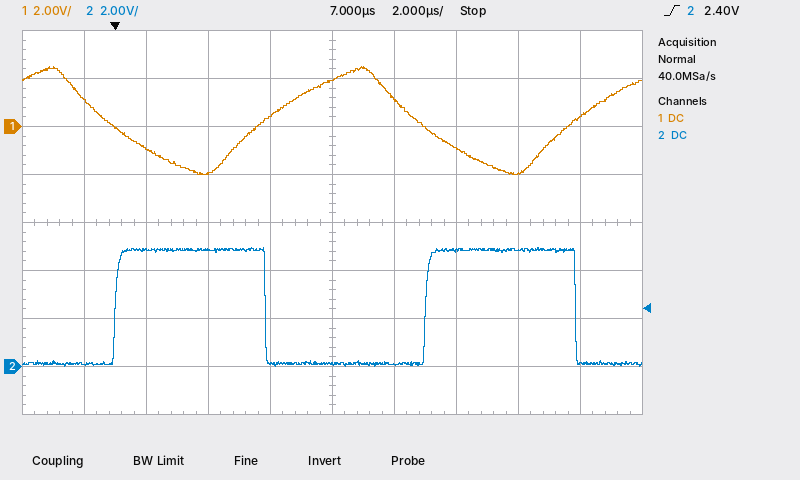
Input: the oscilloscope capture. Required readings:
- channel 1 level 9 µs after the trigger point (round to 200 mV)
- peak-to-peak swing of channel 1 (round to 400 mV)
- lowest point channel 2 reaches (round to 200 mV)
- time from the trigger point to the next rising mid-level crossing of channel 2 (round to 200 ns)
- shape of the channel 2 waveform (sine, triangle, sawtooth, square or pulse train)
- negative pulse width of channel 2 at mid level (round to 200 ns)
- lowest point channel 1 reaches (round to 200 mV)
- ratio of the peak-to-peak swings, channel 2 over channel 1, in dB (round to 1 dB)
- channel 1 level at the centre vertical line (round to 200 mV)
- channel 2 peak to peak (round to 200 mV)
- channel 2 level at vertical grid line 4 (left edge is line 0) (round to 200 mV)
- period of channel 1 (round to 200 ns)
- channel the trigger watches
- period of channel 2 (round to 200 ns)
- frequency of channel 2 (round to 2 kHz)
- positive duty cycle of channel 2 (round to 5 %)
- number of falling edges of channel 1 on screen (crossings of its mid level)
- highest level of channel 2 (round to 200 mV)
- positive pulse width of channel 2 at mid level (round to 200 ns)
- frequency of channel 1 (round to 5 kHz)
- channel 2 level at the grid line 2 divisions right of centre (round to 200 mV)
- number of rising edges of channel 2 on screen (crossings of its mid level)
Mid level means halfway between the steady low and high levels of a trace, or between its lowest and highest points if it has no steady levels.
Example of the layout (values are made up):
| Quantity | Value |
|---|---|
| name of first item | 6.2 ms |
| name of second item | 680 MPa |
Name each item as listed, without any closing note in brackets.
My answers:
| Quantity | Value |
|---|---|
| channel 1 level 9 µs after the trigger point | 1.2 V |
| peak-to-peak swing of channel 1 | 4.4 V |
| lowest point channel 2 reaches | 0.0 V |
| time from the trigger point to the next rising mid-level crossing of channel 2 | 10.0 µs |
| shape of the channel 2 waveform | square |
| negative pulse width of channel 2 at mid level | 5.2 µs |
| lowest point channel 1 reaches | -2.0 V |
| ratio of the peak-to-peak swings, channel 2 over channel 1, in dB | 1 dB |
| channel 1 level at the centre vertical line | 2.0 V |
| channel 2 peak to peak | 5.0 V |
| channel 2 level at vertical grid line 4 (left edge is line 0) | 200 mV |
| period of channel 1 | 10.0 µs |
| channel the trigger watches | channel 2 |
| period of channel 2 | 10.0 µs |
| frequency of channel 2 | 100 kHz |
| positive duty cycle of channel 2 | 50 % |
| number of falling edges of channel 1 on screen | 2 |
| highest level of channel 2 | 5.0 V |
| positive pulse width of channel 2 at mid level | 4.8 µs |
| frequency of channel 1 | 100 kHz |
| channel 2 level at the grid line 2 divisions right of centre | 4.8 V |
| number of rising edges of channel 2 on screen | 2 |
